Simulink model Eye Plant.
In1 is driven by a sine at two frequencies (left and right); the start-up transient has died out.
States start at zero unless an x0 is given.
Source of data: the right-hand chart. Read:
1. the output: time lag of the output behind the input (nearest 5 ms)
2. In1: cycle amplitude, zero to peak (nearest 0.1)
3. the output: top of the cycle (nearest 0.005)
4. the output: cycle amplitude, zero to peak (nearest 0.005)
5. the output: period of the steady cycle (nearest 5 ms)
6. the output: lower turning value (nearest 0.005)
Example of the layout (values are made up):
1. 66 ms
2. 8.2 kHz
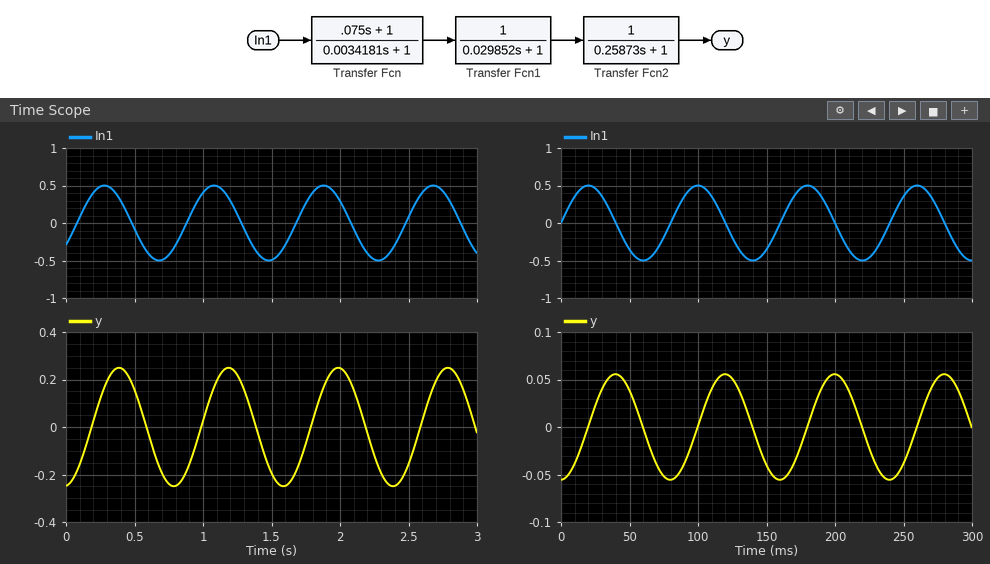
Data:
1. 20 ms
2. 0.5
3. 0.055
4. 0.055
5. 80 ms
6. -0.055
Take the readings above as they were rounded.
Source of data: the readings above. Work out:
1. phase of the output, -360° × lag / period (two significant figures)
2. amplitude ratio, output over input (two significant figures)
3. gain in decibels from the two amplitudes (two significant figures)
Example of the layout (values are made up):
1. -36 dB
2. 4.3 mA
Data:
1. -90°
2. 0.11
3. -19 dB
